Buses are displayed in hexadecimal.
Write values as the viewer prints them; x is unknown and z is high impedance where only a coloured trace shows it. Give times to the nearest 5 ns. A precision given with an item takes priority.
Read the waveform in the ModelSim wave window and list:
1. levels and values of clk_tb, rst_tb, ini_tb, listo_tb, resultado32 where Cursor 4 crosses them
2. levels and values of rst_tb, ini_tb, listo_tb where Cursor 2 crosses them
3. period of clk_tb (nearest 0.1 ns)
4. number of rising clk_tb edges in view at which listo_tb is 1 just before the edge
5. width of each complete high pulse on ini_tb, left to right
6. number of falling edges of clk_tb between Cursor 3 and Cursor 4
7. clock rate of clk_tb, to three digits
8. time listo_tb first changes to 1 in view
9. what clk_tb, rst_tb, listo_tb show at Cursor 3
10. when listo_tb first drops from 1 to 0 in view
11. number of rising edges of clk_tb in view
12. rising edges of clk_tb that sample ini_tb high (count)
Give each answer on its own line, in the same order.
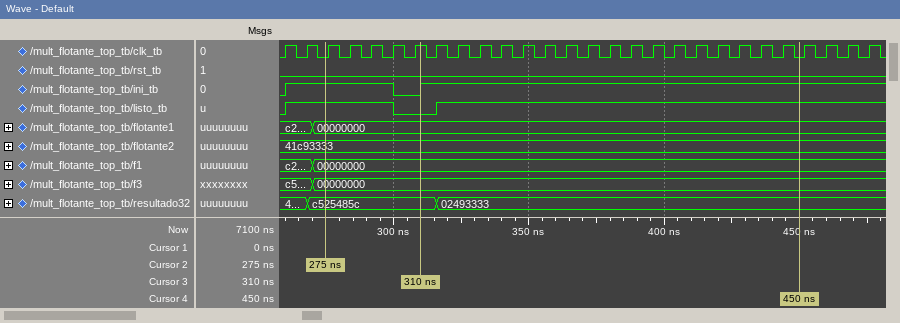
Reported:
clk_tb=0, rst_tb=0, ini_tb=1, listo_tb=1, resultado32=02493333
rst_tb=0, ini_tb=1, listo_tb=1
8 ns
25
40 ns
18
125 MHz
260 ns
clk_tb=1, rst_tb=0, listo_tb=0
300 ns
28
26
